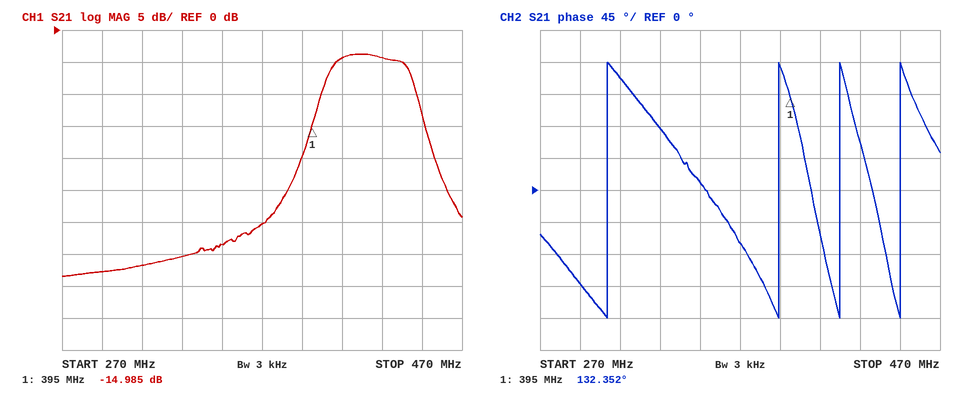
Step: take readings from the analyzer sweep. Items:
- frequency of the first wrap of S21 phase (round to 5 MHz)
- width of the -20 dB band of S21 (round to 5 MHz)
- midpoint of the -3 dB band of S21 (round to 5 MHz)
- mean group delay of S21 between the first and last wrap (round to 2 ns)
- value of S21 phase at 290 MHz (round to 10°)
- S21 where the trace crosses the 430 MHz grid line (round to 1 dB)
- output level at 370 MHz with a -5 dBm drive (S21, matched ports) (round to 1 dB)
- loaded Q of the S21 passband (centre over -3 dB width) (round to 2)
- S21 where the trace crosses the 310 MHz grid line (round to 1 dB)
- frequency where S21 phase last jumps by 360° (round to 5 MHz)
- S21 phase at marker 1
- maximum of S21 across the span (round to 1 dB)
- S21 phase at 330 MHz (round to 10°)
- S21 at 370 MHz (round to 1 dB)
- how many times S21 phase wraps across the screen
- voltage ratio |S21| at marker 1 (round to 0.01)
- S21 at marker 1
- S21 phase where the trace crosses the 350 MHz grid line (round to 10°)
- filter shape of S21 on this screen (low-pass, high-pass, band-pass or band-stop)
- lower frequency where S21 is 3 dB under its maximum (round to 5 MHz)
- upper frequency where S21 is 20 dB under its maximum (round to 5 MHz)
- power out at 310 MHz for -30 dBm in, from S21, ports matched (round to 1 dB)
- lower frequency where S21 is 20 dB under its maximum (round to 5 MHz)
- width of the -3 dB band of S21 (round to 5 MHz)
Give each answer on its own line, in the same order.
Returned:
305 MHz
75 MHz
425 MHz
20 ns
-130°
-4 dB
-35 dBm
10
-37 dB
450 MHz
132.352°
-4 dB
90°
-30 dB
4
0.18
-14.985 dB
10°
band-pass
405 MHz
460 MHz
-67 dBm
385 MHz
40 MHz
